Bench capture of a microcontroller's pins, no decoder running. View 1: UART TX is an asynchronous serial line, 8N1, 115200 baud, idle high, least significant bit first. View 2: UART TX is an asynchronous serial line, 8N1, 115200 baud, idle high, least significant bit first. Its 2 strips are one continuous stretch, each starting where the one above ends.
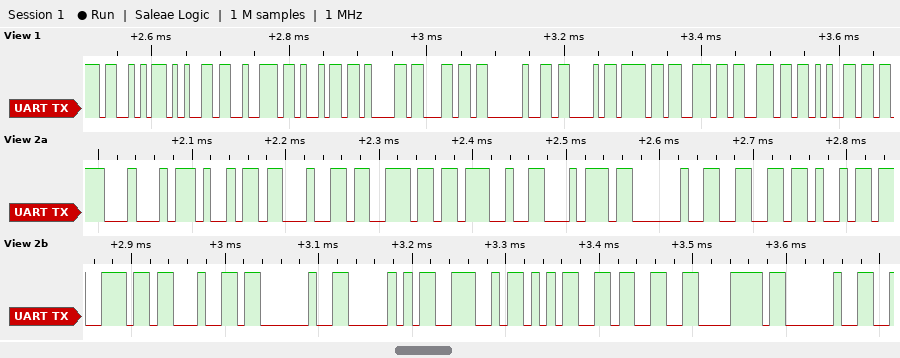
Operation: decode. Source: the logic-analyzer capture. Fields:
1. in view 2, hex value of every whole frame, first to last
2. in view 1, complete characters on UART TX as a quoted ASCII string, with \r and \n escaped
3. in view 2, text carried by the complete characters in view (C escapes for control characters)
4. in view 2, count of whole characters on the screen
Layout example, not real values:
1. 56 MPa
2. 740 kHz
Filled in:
1. 0x44 0x69 0x64 0x6E 0x27 0x74 0x20 0x66 0x69 0x6E 0x64 0x20 0x50 0x4E 0x35 0x33 0x78 0x20
2. "Serial Conne"
3. "Didn't find PN53x "
4. 18
